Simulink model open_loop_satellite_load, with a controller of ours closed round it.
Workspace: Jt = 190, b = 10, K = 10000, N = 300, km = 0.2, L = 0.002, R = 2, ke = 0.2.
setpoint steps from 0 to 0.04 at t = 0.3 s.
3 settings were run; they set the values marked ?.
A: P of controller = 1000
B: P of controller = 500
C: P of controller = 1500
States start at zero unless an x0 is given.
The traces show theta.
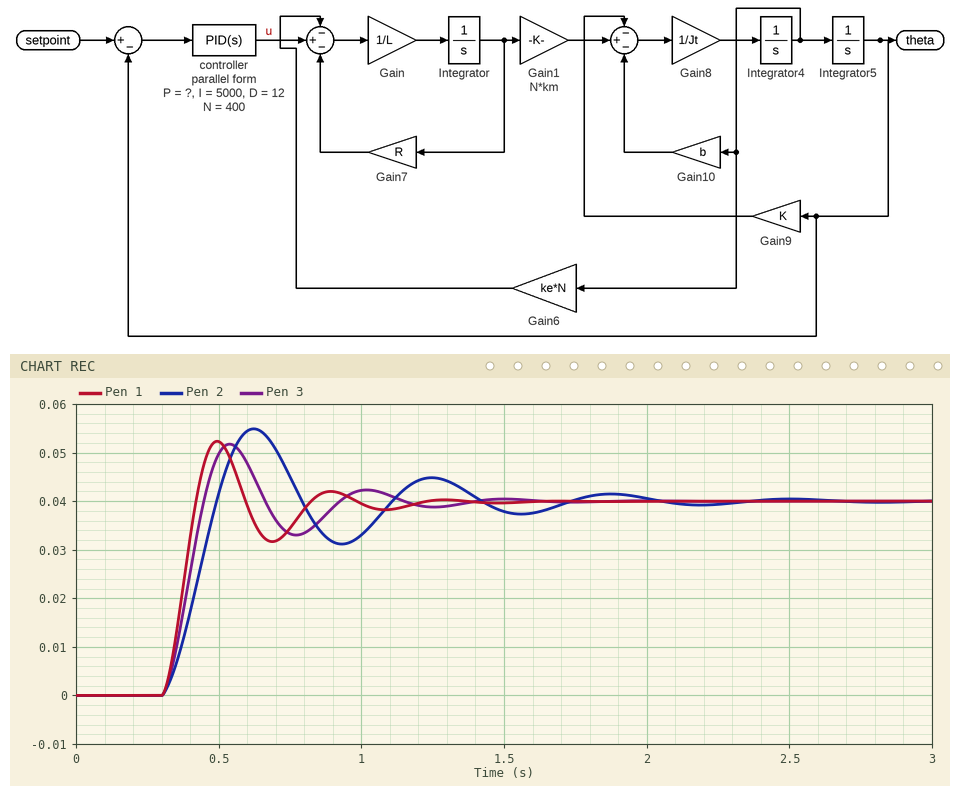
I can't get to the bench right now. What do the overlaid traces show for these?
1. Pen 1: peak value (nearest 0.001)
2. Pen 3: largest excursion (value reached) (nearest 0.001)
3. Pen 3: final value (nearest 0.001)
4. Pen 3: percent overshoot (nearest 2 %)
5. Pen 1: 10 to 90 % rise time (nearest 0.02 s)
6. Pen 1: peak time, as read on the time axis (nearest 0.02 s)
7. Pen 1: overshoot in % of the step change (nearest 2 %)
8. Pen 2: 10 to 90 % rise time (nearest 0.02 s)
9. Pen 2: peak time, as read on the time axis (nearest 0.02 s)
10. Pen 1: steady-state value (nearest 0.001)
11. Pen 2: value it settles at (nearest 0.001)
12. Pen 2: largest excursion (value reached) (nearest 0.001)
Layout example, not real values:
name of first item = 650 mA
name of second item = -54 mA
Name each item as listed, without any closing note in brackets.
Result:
Pen 1: peak value = 0.052
Pen 3: largest excursion (value reached) = 0.052
Pen 3: final value = 0.040
Pen 3: percent overshoot = 30 %
Pen 1: 10 to 90 % rise time = 0.08 s
Pen 1: peak time, as read on the time axis = 0.50 s
Pen 1: overshoot in % of the step change = 30 %
Pen 2: 10 to 90 % rise time = 0.14 s
Pen 2: peak time, as read on the time axis = 0.62 s
Pen 1: steady-state value = 0.040
Pen 2: value it settles at = 0.040
Pen 2: largest excursion (value reached) = 0.055
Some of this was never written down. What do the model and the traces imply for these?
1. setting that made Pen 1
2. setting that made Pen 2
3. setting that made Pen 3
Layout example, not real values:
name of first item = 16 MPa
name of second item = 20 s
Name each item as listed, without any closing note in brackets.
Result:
setting that made Pen 1 = C
setting that made Pen 2 = B
setting that made Pen 3 = A
